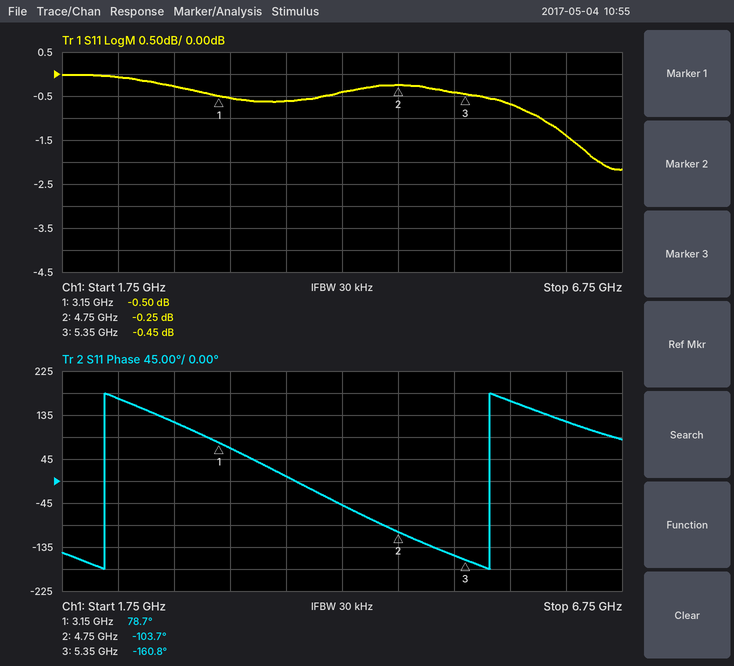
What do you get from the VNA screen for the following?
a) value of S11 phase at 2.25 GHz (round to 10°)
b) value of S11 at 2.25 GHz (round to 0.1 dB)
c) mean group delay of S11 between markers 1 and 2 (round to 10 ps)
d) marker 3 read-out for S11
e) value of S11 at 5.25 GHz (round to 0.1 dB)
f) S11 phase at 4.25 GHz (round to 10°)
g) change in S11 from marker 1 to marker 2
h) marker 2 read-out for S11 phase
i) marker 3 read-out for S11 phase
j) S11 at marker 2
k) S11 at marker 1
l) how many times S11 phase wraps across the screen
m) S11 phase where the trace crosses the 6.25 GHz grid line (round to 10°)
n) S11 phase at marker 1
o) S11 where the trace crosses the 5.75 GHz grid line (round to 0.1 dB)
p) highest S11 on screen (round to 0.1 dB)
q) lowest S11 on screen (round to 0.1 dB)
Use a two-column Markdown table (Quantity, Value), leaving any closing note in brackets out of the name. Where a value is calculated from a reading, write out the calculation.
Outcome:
| Quantity | Value |
|---|---|
| value of S11 phase at 2.25 GHz | 170° |
| value of S11 at 2.25 GHz | -0.1 dB |
| mean group delay of S11 between markers 1 and 2 | −(-103.7° − (78.7°))/(360° × 1.6 GHz) ≈ 317 ps, so 320 ps to the nearest 10 ps |
| marker 3 read-out for S11 | -0.45 dB |
| value of S11 at 5.25 GHz | -0.4 dB |
| S11 phase at 4.25 GHz | -50° |
| change in S11 from marker 1 to marker 2 | -0.25 − (-0.5) = 0.25 dB |
| marker 2 read-out for S11 phase | -103.7° |
| marker 3 read-out for S11 phase | -160.8° |
| S11 at marker 2 | -0.25 dB |
| S11 at marker 1 | -0.50 dB |
| how many times S11 phase wraps across the screen | 2 |
| S11 phase where the trace crosses the 6.25 GHz grid line | 120° |
| S11 phase at marker 1 | 78.7° |
| S11 where the trace crosses the 5.75 GHz grid line | -0.7 dB |
| highest S11 on screen | 0.0 dB |
| lowest S11 on screen | -2.2 dB |
